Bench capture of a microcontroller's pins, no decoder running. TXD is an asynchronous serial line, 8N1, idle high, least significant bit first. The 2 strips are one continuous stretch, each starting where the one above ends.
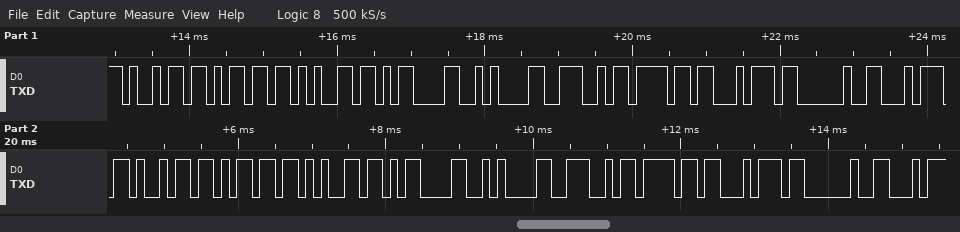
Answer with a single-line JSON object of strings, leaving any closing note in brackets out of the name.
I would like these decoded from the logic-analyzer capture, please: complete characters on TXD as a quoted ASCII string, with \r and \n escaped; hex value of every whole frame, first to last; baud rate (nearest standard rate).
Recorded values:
{"complete characters on TXD as a quoted ASCII string, with \\r and \\n escaped": "\"ime\\r\\nNot time\\r\\nNot \"", "hex value of every whole frame, first to last": "69 6D 65 0D 0A 4E 6F 74 20 74 69 6D 65 0D 0A 4E 6F 74 20", "baud rate": "9600 baud"}
